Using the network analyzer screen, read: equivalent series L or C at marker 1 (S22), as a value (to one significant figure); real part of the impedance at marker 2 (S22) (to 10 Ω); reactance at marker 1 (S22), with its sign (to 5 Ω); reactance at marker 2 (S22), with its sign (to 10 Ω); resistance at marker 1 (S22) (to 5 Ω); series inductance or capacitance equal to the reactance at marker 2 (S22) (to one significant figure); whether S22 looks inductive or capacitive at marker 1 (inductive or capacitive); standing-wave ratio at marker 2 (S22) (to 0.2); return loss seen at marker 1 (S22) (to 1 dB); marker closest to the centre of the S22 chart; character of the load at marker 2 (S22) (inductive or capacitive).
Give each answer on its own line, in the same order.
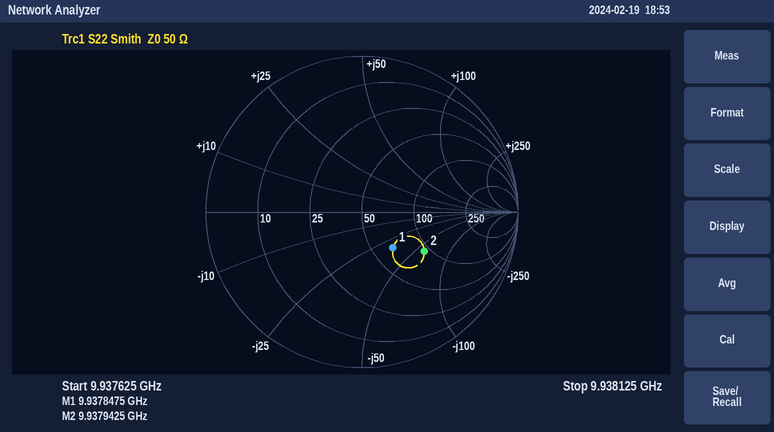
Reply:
500 fF
90 Ω
-35 Ω
-60 Ω
65 Ω
300 fF
capacitive
2.8
10 dB
marker 1
capacitive
